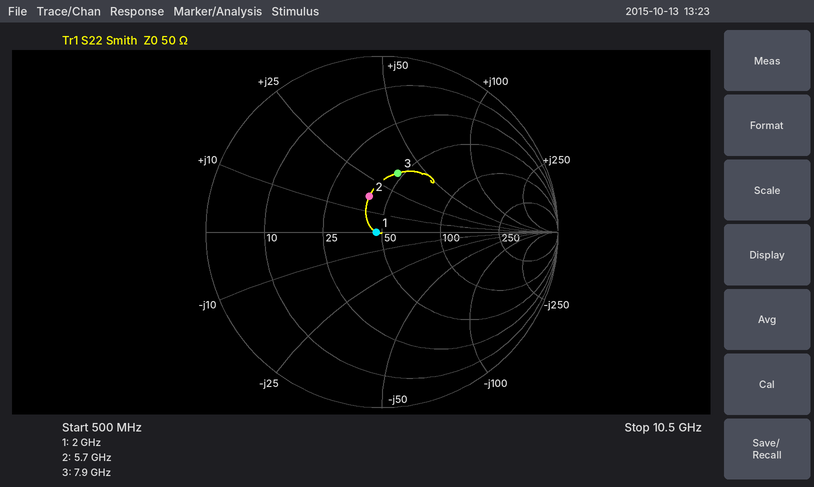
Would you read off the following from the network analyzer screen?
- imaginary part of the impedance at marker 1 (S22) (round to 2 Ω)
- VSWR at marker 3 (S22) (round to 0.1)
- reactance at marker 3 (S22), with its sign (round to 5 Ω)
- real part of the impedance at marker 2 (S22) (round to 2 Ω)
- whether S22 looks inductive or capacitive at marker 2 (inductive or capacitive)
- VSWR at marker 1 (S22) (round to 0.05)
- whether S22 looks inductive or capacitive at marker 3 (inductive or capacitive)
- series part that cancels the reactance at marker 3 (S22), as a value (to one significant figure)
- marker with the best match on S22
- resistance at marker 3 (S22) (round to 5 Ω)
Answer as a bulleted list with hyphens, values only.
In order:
- 0 Ω
- 2.1
- +35 Ω
- 40 Ω
- inductive
- 1.05
- inductive
- 600 fF
- marker 1
- 45 Ω
